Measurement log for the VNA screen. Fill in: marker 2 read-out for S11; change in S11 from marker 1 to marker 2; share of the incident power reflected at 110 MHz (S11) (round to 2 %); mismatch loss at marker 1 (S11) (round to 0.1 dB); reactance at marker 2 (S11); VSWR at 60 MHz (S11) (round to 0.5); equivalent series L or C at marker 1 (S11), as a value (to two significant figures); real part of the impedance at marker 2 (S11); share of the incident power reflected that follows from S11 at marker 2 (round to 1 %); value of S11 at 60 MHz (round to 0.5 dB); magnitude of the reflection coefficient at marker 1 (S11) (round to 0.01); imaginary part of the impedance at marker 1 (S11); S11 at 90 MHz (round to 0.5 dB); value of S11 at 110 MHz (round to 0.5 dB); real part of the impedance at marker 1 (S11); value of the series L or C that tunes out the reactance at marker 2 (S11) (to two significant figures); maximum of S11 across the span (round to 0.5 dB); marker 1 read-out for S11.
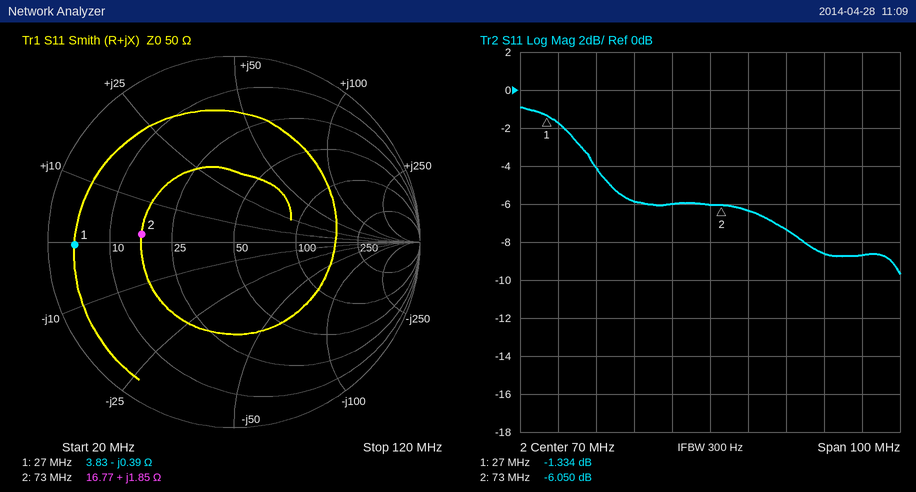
-6.050 dB
-4.716 dB
14 %
5.8 dB
+1.85 Ω
3.0
15 nF
16.77 Ω
25 %
-6.0 dB
0.86
-0.39 Ω
-7.5 dB
-8.5 dB
3.83 Ω
1.2 nF
-1.0 dB
-1.334 dB
